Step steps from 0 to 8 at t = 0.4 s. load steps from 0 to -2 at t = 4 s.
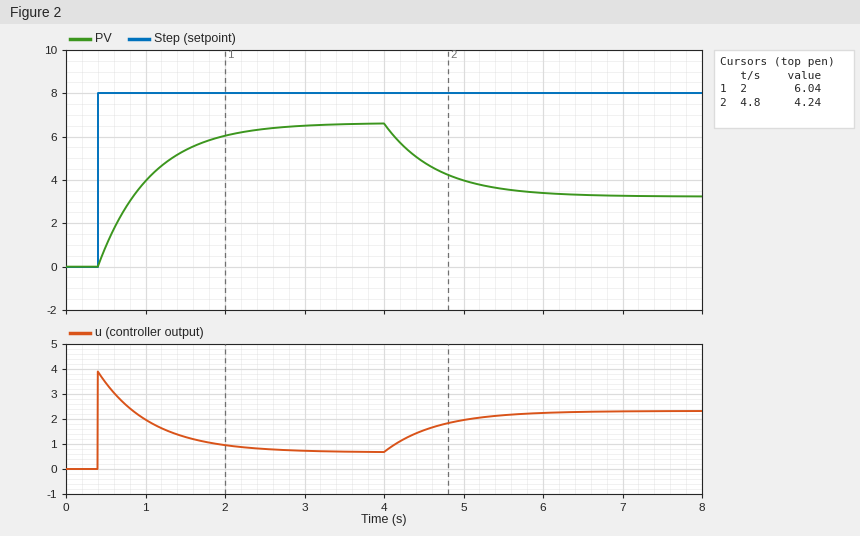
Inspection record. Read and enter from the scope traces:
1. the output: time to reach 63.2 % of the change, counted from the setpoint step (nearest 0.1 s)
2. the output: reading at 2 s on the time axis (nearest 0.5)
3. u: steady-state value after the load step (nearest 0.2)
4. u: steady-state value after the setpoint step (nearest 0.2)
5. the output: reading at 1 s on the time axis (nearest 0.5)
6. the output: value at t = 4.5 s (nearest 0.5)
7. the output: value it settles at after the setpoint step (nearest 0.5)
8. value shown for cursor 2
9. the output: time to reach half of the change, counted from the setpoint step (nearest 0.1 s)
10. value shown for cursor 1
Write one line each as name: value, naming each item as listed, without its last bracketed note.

the output: time to reach 63.2 % of the change, counted from the setpoint step: 0.7 s
the output: reading at 2 s on the time axis: 6.0
u: steady-state value after the load step: 2.4
u: steady-state value after the setpoint step: 0.6
the output: reading at 1 s on the time axis: 4.0
the output: value at t = 4.5 s: 5.0
the output: value it settles at after the setpoint step: 6.5
value shown for cursor 2: 4.24
the output: time to reach half of the change, counted from the setpoint step: 0.5 s
value shown for cursor 1: 6.04
